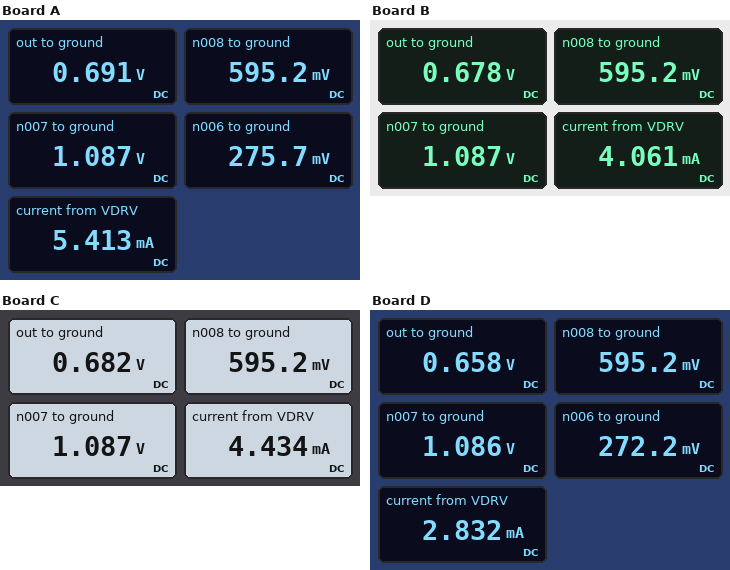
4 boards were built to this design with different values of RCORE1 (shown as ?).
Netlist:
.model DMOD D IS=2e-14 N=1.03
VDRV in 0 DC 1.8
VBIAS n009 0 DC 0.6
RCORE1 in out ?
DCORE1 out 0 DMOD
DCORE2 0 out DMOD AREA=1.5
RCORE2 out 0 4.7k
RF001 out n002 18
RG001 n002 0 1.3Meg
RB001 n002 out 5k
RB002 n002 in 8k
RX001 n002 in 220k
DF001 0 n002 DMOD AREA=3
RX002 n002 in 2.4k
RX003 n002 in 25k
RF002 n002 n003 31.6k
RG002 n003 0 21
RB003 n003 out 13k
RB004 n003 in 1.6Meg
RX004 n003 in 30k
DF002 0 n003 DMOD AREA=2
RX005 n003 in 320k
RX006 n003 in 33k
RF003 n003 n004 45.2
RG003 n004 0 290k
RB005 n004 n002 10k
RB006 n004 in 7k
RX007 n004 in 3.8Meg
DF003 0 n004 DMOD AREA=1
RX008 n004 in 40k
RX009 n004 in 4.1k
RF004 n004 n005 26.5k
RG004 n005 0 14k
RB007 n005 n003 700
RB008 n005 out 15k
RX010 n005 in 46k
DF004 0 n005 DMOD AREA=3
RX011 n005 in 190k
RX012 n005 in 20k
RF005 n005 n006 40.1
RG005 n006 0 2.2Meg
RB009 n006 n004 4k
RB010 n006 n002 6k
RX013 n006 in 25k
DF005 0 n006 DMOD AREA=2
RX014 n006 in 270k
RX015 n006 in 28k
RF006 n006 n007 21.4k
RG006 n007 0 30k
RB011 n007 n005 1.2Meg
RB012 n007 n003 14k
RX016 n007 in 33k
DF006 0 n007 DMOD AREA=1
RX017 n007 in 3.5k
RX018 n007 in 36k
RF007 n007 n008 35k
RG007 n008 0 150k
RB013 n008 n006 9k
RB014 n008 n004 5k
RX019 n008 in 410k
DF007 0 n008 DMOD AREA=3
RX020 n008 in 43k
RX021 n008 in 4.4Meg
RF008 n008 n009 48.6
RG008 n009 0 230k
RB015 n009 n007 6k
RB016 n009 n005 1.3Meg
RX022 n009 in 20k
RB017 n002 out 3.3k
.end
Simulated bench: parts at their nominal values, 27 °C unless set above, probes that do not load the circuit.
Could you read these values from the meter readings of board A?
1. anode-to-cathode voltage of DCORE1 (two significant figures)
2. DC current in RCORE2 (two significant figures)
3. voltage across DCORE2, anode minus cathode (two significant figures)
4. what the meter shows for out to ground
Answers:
690 mV
150 µA
-690 mV
0.691 V
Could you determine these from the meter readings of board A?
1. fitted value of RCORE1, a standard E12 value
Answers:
330 Ω
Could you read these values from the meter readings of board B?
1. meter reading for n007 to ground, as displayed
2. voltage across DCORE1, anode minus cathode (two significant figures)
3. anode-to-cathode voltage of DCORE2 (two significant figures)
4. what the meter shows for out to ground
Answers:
1.087 V
680 mV
-680 mV
0.678 V
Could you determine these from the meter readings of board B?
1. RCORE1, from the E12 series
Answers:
560 Ω
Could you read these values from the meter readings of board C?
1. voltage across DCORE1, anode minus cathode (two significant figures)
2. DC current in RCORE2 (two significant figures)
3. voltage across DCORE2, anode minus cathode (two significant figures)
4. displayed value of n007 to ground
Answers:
680 mV
150 µA
-680 mV
1.087 V
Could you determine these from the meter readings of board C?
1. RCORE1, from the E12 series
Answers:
470 Ω
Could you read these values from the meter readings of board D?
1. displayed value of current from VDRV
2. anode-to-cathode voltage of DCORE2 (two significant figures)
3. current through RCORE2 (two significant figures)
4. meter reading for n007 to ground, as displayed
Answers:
2.832 mA
-660 mV
140 µA
1.086 V
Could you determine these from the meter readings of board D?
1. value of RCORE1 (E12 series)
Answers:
1.5 kΩ
